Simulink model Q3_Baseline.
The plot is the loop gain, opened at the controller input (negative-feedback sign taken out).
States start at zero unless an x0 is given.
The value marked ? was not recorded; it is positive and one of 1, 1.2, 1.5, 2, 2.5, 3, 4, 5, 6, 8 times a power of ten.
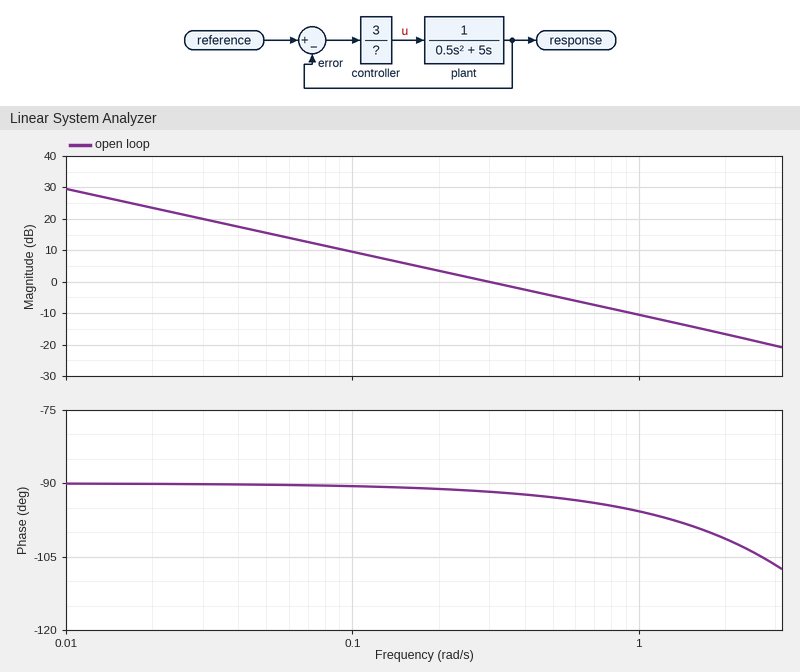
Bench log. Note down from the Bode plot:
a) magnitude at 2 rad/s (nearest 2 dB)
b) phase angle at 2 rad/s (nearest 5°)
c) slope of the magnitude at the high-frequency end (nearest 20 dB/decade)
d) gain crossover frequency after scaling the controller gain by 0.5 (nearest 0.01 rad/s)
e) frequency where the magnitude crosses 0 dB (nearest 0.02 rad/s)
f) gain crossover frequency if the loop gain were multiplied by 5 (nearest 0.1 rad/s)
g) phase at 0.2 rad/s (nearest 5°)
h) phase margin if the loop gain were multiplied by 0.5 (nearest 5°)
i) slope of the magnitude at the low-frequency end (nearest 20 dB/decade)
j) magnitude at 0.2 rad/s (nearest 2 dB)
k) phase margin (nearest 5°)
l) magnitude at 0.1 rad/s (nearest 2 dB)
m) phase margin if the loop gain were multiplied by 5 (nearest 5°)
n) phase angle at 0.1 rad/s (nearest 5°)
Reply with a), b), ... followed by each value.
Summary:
a) -16 dB
b) -100°
c) -20 dB/decade
d) 0.15 rad/s
e) 0.30 rad/s
f) 1.5 rad/s
g) -90°
h) 90°
i) -20 dB/decade
j) 4 dB
k) 90°
l) 10 dB
m) 80°
n) -90°
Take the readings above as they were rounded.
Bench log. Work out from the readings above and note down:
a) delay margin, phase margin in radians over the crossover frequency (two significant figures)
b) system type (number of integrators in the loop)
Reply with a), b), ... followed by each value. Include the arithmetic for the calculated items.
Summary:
a) 90 × π / 180 / 0.3 = 5.2 s
b) 1
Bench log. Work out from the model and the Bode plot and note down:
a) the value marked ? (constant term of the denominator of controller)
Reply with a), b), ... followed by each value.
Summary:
a) 2
